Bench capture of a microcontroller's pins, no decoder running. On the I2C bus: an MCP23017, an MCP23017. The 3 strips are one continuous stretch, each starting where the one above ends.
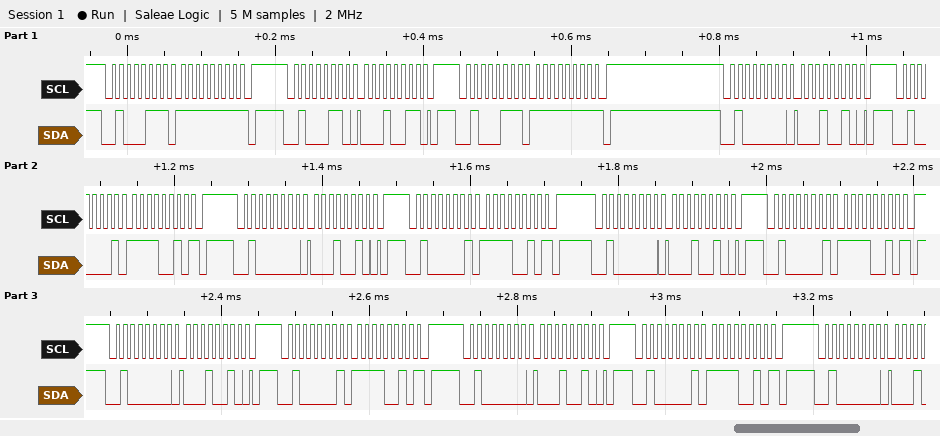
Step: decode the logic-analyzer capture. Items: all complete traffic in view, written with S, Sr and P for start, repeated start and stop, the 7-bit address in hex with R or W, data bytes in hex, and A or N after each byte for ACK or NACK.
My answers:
S 23R A FF N P S 23W A 13 A P S 23R A FF N P S 20W A 12 A P S 20R A F2 N P S 20W A 12 A P S 20R A F2 N P S 20W A 12 A P S 20R A F2 N P S 20W A 12 A P S 20R A F2 N P S 20W A 12 A P S 20R A F2 N P S 20W A
